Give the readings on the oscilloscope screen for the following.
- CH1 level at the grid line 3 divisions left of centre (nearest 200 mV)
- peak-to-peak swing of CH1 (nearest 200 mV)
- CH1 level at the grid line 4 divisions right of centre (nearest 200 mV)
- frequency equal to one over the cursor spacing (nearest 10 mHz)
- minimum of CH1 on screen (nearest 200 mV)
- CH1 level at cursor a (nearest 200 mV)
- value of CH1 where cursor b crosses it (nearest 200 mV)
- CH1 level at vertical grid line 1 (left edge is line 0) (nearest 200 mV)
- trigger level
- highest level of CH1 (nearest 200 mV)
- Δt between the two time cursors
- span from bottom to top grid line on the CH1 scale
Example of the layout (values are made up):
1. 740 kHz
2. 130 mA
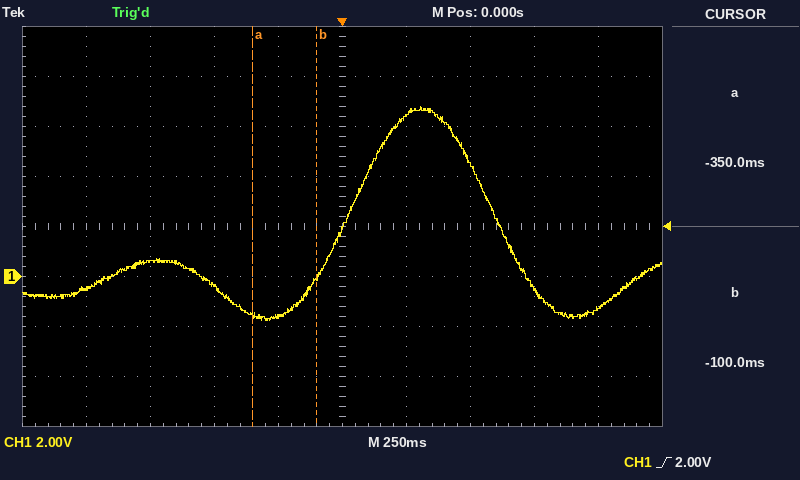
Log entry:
1. 600 mV
2. 8.6 V
3. -1.2 V
4. 4.00 Hz
5. -1.8 V
6. -1.6 V
7. 0.0 V
8. -400 mV
9. 2.00 V
10. 6.8 V
11. 250 ms
12. 16 V
